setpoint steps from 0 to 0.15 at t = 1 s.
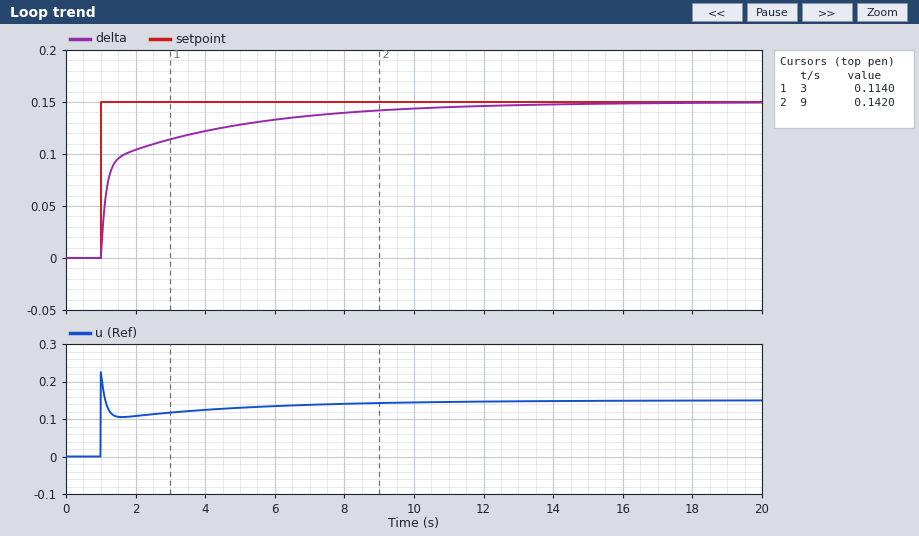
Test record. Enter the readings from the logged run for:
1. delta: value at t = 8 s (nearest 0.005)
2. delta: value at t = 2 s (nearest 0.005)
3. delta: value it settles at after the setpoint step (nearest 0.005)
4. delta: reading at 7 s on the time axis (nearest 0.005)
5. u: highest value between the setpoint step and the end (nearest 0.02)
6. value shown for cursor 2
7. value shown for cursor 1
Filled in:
0.140
0.105
0.150
0.135
0.22
0.1420
0.1140
